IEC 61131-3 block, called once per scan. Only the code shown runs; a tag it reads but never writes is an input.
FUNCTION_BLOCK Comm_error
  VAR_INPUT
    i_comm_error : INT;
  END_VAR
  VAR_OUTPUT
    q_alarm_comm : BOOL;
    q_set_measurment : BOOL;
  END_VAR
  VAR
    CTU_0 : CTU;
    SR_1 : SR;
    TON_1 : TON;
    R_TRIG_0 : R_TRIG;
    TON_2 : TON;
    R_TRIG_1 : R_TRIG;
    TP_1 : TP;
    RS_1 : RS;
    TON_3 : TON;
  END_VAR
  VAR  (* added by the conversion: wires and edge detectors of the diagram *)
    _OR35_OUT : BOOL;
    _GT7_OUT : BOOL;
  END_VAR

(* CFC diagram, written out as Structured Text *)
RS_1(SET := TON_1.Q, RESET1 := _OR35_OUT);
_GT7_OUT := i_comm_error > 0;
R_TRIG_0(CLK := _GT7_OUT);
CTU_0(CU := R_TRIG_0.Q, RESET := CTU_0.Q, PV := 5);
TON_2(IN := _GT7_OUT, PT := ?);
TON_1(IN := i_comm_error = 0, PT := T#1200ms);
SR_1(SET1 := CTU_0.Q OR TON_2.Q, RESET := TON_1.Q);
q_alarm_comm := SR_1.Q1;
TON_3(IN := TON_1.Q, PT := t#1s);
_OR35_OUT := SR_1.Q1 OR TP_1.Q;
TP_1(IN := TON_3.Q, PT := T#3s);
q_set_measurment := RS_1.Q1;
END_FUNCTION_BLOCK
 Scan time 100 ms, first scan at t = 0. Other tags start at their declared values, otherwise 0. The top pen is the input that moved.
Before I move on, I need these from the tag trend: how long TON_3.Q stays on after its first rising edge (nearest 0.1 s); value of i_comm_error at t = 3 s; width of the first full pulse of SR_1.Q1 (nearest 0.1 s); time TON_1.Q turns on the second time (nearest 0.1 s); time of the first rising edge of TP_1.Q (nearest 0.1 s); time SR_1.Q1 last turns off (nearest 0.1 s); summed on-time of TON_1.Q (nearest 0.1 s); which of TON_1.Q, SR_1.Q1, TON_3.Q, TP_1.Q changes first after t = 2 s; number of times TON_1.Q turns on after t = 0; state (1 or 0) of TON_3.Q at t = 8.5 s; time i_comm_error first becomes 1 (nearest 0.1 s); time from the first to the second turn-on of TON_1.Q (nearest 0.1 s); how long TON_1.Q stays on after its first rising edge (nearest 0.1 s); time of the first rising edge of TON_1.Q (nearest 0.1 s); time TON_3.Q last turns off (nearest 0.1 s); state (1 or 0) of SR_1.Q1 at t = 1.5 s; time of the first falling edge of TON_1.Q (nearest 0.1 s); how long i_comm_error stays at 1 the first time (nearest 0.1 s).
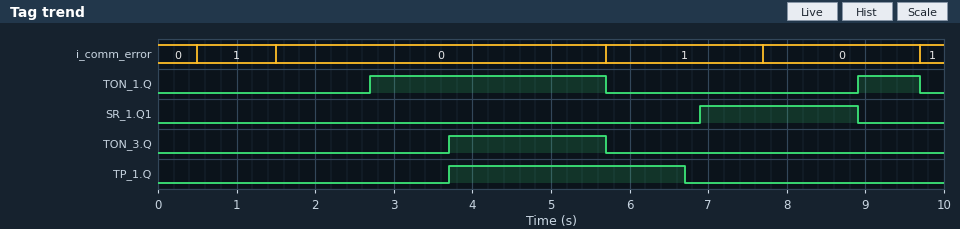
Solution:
2.0 s
0
2.0 s
8.9 s
3.7 s
8.9 s
3.8 s
TON_1.Q
2
0
0.5 s
6.2 s
3.0 s
2.7 s
5.7 s
0
5.7 s
1.0 s
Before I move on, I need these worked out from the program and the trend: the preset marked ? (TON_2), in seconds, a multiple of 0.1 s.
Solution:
1.2 s
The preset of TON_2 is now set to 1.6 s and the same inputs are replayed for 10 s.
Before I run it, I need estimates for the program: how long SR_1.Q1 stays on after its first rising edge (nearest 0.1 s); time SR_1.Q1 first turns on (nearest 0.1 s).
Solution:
1.6 s
7.3 s
